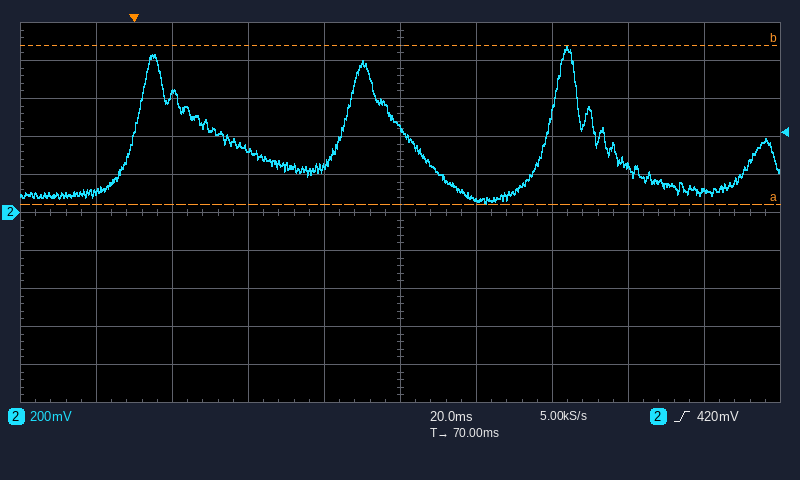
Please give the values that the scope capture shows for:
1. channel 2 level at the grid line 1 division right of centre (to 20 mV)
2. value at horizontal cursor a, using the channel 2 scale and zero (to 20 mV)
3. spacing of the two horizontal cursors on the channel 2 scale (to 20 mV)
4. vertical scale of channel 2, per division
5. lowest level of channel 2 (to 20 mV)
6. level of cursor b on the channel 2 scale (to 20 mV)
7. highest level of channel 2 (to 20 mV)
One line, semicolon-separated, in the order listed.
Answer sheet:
60 mV; 40 mV; 840 mV; 200 mV; 40 mV; 880 mV; 880 mV
